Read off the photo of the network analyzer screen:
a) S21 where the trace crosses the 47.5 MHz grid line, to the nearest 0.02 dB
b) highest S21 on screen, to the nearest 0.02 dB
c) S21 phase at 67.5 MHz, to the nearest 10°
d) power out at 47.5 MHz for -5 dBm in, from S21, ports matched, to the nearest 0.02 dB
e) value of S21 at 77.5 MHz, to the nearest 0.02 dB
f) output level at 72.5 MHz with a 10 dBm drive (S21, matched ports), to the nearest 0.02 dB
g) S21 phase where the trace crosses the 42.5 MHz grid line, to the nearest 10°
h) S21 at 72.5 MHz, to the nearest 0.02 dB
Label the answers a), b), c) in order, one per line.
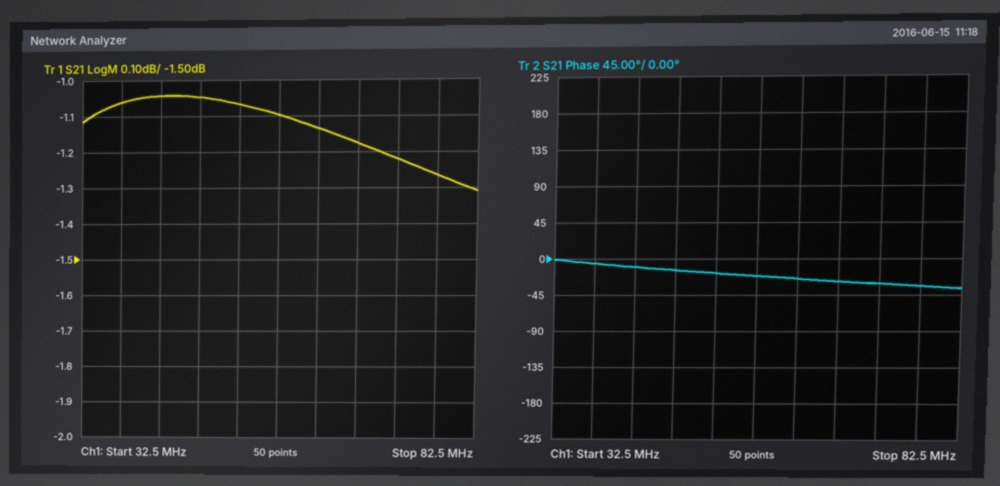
a) -1.04 dB
b) -1.04 dB
c) -30°
d) -6.04 dBm
e) -1.26 dB
f) 8.78 dBm
g) -10°
h) -1.22 dB
